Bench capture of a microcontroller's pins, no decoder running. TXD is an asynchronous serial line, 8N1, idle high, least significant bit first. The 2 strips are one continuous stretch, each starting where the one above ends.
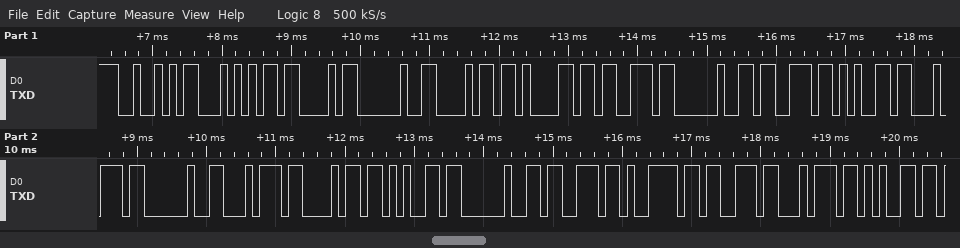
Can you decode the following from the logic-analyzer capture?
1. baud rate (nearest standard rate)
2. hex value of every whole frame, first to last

9600 baud
0x52 0x54 0x43 0x20 0x68 0x61 0x73 0x20 0x73 0x65 0x74 0x20 0x74 0x68 0x65 0x20 0x73 0x79 0x73 0x74 0x65
